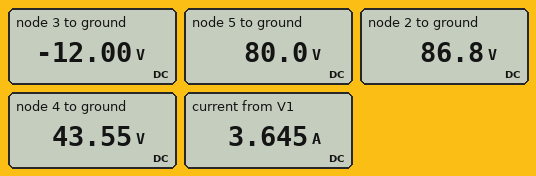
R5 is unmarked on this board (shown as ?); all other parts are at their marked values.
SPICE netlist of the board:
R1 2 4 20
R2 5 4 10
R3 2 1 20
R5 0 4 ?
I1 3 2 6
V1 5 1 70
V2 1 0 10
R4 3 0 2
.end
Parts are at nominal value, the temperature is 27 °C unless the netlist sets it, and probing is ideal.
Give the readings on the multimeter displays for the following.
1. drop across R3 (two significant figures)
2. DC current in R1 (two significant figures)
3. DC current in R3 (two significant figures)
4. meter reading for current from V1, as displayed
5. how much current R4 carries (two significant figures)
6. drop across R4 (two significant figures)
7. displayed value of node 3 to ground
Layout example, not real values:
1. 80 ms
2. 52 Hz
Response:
1. 77 V
2. 2.2 A
3. 3.8 A
4. 3.645 A
5. 6.0 A
6. 12 V
7. -12.00 V
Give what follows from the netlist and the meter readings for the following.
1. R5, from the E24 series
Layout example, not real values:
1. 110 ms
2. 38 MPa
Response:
1. 7.5 Ω
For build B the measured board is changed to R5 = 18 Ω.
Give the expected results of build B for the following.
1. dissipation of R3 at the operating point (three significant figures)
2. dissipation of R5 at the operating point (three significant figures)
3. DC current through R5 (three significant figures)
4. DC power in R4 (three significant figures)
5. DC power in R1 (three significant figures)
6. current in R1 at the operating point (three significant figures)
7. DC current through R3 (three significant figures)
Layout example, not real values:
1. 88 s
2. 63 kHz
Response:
1. 371 W
2. 216 W
3. 3.46 A
4. 72.0 W
5. 57.3 W
6. 1.69 A
7. 4.31 A
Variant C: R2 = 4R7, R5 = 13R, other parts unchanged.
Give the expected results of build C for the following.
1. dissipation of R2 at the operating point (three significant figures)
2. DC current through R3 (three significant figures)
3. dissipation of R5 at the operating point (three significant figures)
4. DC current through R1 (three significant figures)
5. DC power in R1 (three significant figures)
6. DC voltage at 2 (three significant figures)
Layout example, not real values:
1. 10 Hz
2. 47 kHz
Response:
1. 51.7 W
2. 4.36 A
3. 319 W
4. 1.64 A
5. 53.8 W
6. 97.2 V
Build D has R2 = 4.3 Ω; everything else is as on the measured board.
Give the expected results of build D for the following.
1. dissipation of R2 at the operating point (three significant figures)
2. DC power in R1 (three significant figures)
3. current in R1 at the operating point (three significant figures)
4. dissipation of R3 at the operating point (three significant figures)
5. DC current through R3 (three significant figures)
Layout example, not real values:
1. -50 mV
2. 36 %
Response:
1. 135 W
2. 68.6 W
3. 1.85 A
4. 344 W
5. 4.15 A
